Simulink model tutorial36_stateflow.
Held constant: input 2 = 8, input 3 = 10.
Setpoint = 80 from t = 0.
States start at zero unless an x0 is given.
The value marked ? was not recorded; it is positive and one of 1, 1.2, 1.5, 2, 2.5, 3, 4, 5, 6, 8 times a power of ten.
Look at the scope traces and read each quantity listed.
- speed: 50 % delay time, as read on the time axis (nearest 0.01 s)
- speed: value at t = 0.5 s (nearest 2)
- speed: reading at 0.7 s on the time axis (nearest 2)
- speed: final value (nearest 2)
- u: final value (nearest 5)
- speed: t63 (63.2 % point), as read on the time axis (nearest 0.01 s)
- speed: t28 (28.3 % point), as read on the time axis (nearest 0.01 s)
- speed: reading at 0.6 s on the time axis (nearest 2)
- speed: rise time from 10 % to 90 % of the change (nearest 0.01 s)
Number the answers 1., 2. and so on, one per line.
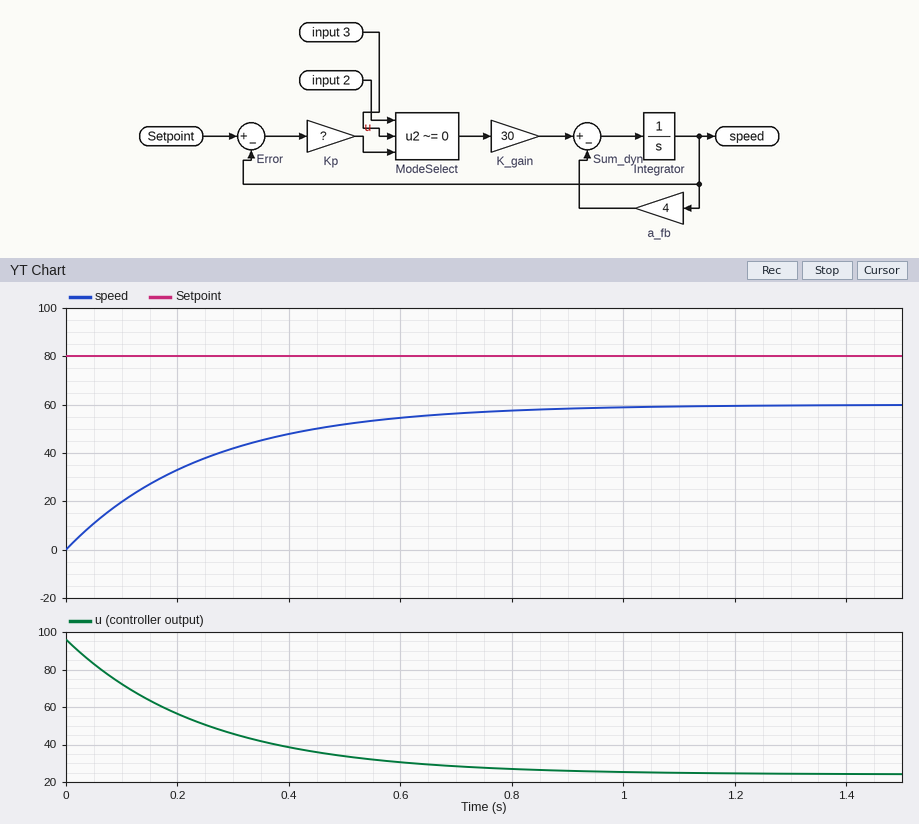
1. 0.17 s
2. 52
3. 56
4. 60
5. 25
6. 0.25 s
7. 0.08 s
8. 54
9. 0.55 s
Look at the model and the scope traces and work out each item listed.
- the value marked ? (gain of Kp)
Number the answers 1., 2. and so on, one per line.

1. 1.2
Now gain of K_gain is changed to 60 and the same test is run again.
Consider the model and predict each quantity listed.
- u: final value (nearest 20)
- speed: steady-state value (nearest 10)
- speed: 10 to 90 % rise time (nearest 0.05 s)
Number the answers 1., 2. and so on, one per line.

1. -40
2. 120
3. 0.55 s
